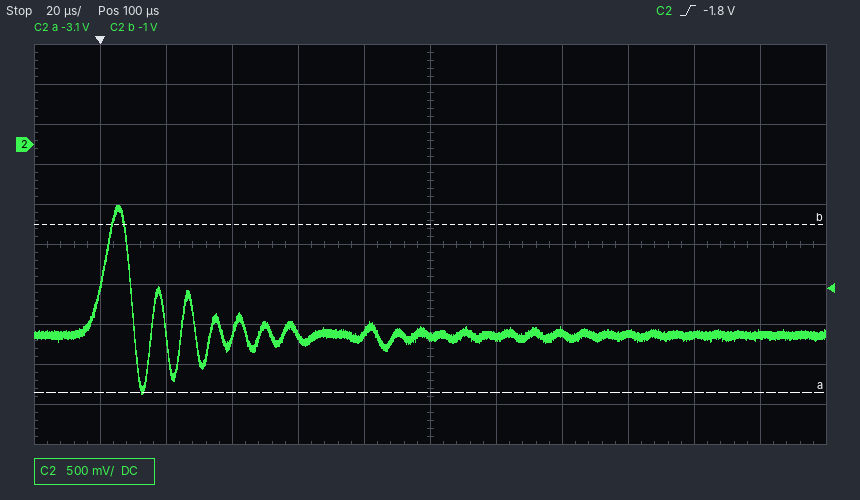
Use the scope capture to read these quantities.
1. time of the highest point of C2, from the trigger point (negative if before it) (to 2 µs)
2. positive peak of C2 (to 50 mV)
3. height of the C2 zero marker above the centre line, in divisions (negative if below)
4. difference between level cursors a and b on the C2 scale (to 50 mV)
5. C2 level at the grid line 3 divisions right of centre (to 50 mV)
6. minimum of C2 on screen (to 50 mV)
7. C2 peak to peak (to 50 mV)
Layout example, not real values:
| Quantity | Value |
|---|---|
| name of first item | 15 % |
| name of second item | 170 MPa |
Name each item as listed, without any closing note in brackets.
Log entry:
| Quantity | Value |
|---|---|
| time of the highest point of C2, from the trigger point (negative if before it) | +6 µs |
| positive peak of C2 | -750 mV |
| height of the C2 zero marker above the centre line, in divisions | +2.5 div |
| difference between level cursors a and b on the C2 scale | 2.10 V |
| C2 level at the grid line 3 divisions right of centre | -2.35 V |
| minimum of C2 on screen | -3.10 V |
| C2 peak to peak | 2.35 V |
